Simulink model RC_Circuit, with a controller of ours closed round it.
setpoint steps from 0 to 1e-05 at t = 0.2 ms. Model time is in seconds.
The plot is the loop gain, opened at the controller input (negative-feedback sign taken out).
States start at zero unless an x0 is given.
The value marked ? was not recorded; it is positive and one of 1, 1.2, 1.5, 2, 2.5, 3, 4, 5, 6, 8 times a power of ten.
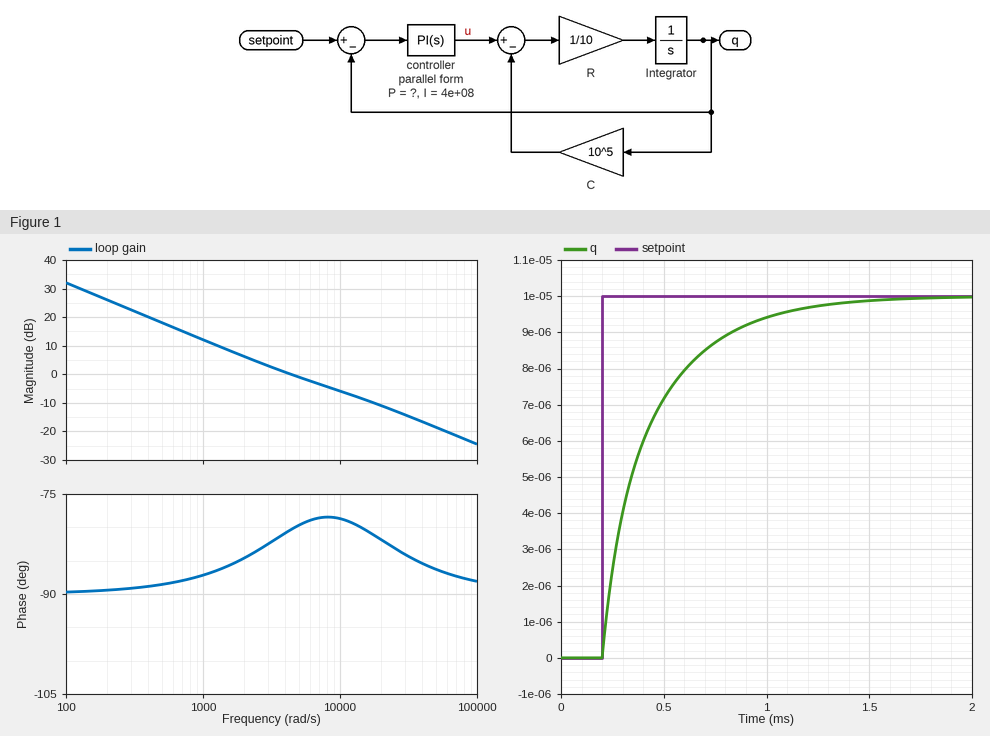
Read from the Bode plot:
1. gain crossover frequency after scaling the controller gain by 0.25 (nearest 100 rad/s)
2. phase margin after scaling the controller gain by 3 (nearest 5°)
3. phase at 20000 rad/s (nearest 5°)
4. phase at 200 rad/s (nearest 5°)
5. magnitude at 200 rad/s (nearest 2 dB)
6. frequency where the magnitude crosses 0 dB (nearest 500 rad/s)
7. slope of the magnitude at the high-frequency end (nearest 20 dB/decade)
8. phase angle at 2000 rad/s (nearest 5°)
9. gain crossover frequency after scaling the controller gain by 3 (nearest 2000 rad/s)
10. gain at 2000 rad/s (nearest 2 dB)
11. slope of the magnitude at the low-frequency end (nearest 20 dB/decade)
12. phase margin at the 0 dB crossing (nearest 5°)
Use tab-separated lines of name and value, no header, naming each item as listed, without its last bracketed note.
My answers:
gain crossover frequency after scaling the controller gain by 0.25	1000 rad/s
phase margin after scaling the controller gain by 3	100°
phase at 20000 rad/s	-80°
phase at 200 rad/s	-90°
magnitude at 200 rad/s	26 dB
frequency where the magnitude crosses 0 dB	4500 rad/s
slope of the magnitude at the high-frequency end	-20 dB/decade
phase angle at 2000 rad/s	-85°
gain crossover frequency after scaling the controller gain by 3	16000 rad/s
gain at 2000 rad/s	6 dB
slope of the magnitude at the low-frequency end	-20 dB/decade
phase margin at the 0 dB crossing	100°
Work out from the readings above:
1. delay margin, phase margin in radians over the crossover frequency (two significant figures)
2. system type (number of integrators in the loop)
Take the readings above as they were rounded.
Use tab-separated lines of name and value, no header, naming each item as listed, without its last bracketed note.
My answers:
delay margin, phase margin in radians over the crossover frequency	0.00039 s
system type	1
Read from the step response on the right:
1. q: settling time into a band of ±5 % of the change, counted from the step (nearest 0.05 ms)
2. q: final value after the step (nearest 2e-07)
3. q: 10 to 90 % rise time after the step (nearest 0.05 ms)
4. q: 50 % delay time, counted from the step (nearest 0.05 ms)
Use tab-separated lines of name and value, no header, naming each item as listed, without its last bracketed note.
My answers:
q: settling time into a band of ±5 % of the change, counted from the step	0.85 ms
q: final value after the step	0.0000100
q: 10 to 90 % rise time after the step	0.60 ms
q: 50 % delay time, counted from the step	0.15 ms
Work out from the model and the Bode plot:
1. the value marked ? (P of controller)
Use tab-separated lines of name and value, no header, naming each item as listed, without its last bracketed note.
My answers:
the value marked ?	60000
